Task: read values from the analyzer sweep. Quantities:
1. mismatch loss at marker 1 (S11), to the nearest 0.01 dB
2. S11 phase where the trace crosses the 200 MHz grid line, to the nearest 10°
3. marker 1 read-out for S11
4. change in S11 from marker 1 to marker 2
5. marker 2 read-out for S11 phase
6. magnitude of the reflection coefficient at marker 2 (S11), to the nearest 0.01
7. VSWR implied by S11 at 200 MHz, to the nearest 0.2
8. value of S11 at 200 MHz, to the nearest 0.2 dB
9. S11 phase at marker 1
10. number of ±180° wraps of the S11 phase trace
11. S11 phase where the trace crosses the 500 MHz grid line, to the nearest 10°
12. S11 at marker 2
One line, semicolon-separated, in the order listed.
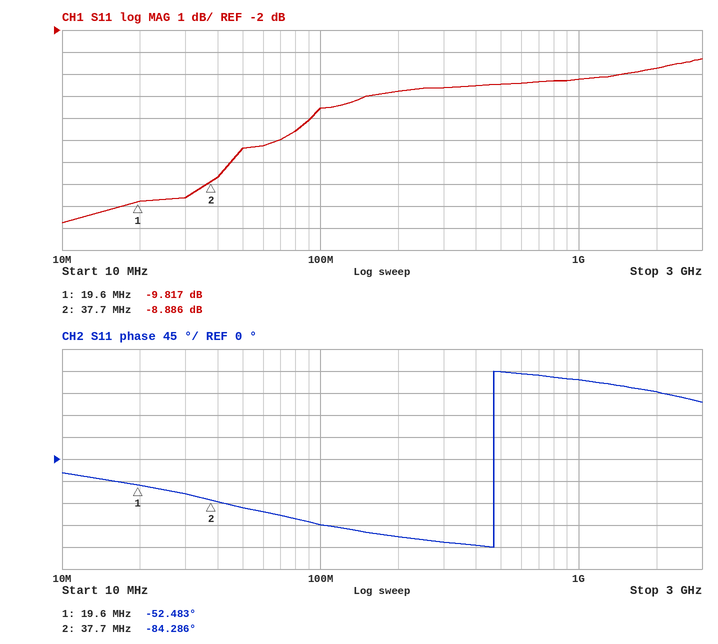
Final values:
0.48 dB; -160°; -9.817 dB; 0.931 dB; -84.286°; 0.36; 3.8; -4.8 dB; -52.483°; 1; 180°; -8.886 dB
